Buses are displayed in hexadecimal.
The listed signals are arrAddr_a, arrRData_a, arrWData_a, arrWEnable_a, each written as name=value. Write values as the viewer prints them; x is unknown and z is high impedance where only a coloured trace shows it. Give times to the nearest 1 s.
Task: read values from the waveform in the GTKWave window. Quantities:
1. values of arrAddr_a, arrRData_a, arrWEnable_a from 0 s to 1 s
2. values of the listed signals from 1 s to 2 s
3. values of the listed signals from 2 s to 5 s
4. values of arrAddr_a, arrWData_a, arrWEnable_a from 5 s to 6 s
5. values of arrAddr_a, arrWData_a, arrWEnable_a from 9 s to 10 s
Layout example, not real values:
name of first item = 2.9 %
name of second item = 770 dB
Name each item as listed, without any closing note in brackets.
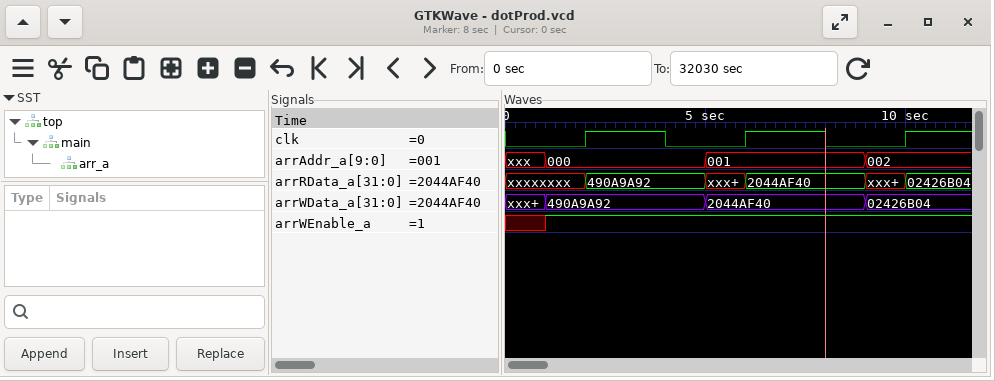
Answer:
values of arrAddr_a, arrRData_a, arrWEnable_a from 0 s to 1 s = arrAddr_a=xxx, arrRData_a=xxxxxxxx, arrWEnable_a=x
values of the listed signals from 1 s to 2 s = arrAddr_a=000, arrRData_a=xxxxxxxx, arrWData_a=490A9A92, arrWEnable_a=1
values of the listed signals from 2 s to 5 s = arrAddr_a=000, arrRData_a=490A9A92, arrWData_a=490A9A92, arrWEnable_a=1
values of arrAddr_a, arrWData_a, arrWEnable_a from 5 s to 6 s = arrAddr_a=001, arrWData_a=2044AF40, arrWEnable_a=1
values of arrAddr_a, arrWData_a, arrWEnable_a from 9 s to 10 s = arrAddr_a=002, arrWData_a=02426B04, arrWEnable_a=1
